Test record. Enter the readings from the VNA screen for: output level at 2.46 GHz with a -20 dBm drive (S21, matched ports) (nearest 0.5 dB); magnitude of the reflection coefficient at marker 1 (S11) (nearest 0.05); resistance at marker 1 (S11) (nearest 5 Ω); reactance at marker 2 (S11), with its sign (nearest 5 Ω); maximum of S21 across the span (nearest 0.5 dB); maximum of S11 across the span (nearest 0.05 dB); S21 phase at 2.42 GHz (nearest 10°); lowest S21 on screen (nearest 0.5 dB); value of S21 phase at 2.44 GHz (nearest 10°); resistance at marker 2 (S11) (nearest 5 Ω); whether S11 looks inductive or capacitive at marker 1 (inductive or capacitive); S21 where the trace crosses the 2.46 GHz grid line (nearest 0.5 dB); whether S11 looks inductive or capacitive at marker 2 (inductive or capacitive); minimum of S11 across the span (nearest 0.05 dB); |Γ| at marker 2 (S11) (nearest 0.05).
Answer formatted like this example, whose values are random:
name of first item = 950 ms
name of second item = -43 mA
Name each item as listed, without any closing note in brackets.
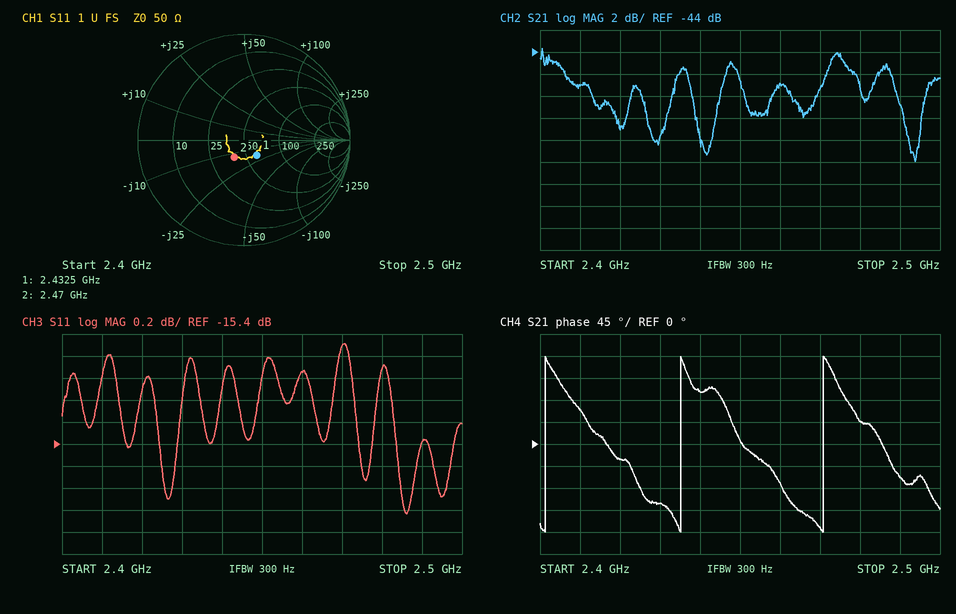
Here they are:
output level at 2.46 GHz with a -20 dBm drive (S21, matched ports) = -67.0 dBm
magnitude of the reflection coefficient at marker 1 (S11) = 0.20
resistance at marker 1 (S11) = 60 Ω
reactance at marker 2 (S11), with its sign = -15 Ω
maximum of S21 across the span = -43.5 dB
maximum of S11 across the span = -14.50 dB
S21 phase at 2.42 GHz = -30°
lowest S21 on screen = -54.0 dB
value of S21 phase at 2.44 GHz = 110°
resistance at marker 2 (S11) = 40 Ω
whether S11 looks inductive or capacitive at marker 1 = capacitive
S21 where the trace crosses the 2.46 GHz grid line = -47.0 dB
whether S11 looks inductive or capacitive at marker 2 = capacitive
minimum of S11 across the span = -16.05 dB
|Γ| at marker 2 (S11) = 0.20
